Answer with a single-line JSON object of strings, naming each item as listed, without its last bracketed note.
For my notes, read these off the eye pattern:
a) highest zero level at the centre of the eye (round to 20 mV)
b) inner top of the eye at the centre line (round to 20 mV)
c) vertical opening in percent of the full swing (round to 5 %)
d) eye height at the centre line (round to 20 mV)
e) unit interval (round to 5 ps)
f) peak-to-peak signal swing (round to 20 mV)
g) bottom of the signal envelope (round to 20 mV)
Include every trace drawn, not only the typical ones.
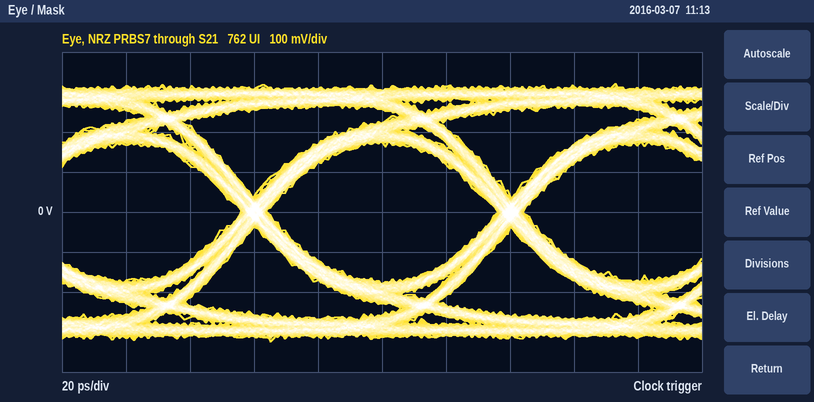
{"highest zero level at the centre of the eye": "-180 mV", "inner top of the eye at the centre line": "180 mV", "vertical opening in percent of the full swing": "55 %", "eye height at the centre line": "360 mV", "unit interval": "80 ps", "peak-to-peak signal swing": "640 mV", "bottom of the signal envelope": "-320 mV"}
